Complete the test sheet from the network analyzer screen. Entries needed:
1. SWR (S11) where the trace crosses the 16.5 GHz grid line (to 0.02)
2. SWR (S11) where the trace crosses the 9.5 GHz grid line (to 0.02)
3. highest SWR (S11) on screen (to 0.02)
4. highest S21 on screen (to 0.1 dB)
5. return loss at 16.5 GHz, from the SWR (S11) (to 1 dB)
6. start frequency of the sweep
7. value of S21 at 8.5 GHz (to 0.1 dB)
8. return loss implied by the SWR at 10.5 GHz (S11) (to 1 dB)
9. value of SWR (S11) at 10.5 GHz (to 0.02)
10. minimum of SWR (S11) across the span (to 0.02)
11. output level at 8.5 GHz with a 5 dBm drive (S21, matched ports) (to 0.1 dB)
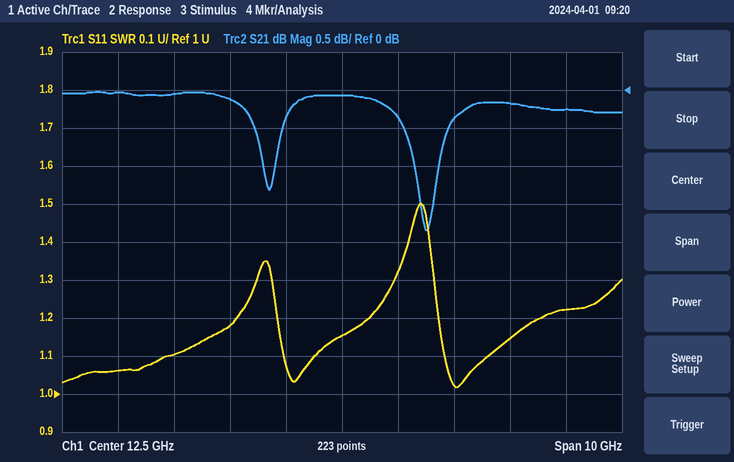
1.22
1.10
1.50
0.0 dB
20 dB
7.5 GHz
0.0 dB
22 dB
1.18
1.02
5.0 dBm
